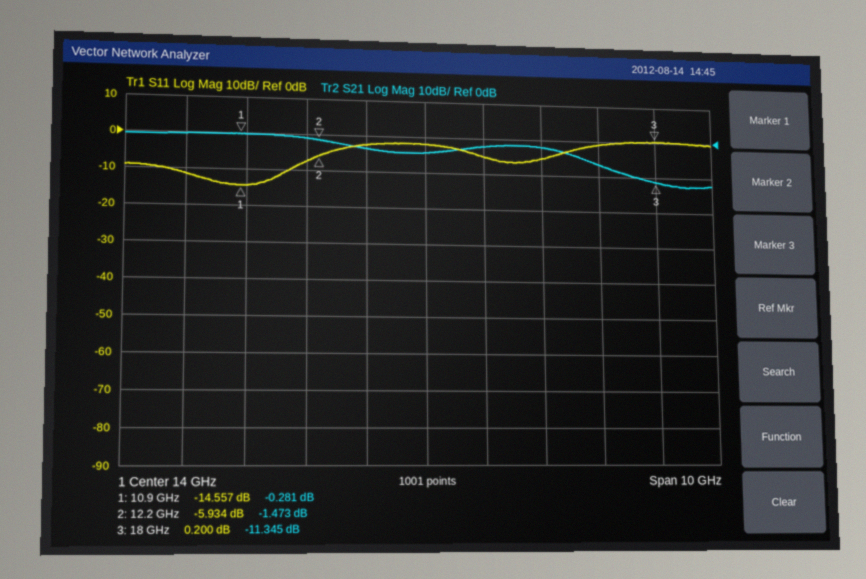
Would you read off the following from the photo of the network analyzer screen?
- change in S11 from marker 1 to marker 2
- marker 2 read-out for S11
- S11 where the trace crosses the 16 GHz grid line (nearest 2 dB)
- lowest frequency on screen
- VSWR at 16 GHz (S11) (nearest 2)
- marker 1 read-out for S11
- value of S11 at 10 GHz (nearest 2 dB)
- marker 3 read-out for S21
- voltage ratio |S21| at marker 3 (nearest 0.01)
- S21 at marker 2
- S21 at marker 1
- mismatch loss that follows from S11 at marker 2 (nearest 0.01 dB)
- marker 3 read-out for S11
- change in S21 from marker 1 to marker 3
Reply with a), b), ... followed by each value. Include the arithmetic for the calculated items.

a) -5.934 − (-14.557) = 8.623 dB
b) -5.934 dB
c) -6 dB
d) 9 GHz
e) |Γ| = 10^(-6/20) = 0.5012; VSWR = (1 + 0.5012)/(1 − 0.5012) ≈ 3.01, so 4 to the nearest 2
f) -14.557 dB
g) -12 dB
h) -11.345 dB
i) 10^(-11.345/20) ≈ 0.27
j) -1.473 dB
k) -0.281 dB
l) −10 log10(1 − 10^(-5.934/10)) ≈ 1.28 dB
m) 0.200 dB
n) -11.345 − (-0.281) = -11.064 dB
